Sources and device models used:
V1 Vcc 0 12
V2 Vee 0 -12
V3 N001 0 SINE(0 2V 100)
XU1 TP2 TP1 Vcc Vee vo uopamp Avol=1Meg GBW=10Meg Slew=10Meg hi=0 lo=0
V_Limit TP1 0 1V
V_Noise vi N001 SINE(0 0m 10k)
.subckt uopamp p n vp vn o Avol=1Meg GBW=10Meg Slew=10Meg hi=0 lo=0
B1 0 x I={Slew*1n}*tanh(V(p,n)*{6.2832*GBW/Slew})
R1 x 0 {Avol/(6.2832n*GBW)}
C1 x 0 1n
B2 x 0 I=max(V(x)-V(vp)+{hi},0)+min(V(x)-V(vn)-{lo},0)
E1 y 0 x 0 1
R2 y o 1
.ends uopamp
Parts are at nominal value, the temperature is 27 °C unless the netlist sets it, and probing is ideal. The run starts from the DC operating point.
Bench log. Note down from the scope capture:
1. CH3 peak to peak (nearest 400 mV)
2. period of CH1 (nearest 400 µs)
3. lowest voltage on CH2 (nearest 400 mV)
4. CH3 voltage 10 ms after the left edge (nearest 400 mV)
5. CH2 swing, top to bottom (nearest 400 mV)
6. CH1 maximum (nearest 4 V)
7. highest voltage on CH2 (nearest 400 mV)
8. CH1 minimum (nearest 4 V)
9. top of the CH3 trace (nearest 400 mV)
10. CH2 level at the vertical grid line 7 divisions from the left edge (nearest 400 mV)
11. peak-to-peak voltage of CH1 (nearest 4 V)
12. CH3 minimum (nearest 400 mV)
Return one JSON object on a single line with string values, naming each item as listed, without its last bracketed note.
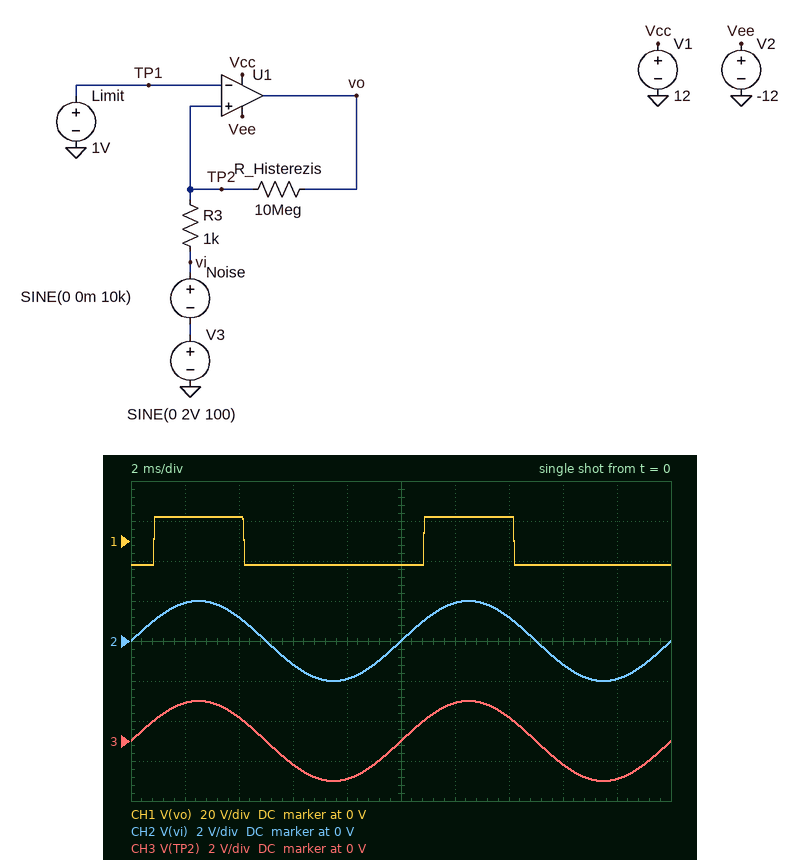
{"CH3 peak to peak": "4.0 V", "period of CH1": "10.0 ms", "lowest voltage on CH2": "-2.0 V", "CH3 voltage 10 ms after the left edge": "0 V", "CH2 swing, top to bottom": "4.0 V", "CH1 maximum": "12 V", "highest voltage on CH2": "2.0 V", "CH1 minimum": "-12 V", "top of the CH3 trace": "2.0 V", "CH2 level at the vertical grid line 7 divisions from the left edge": "1.2 V", "peak-to-peak voltage of CH1": "24 V", "CH3 minimum": "-2.0 V"}
